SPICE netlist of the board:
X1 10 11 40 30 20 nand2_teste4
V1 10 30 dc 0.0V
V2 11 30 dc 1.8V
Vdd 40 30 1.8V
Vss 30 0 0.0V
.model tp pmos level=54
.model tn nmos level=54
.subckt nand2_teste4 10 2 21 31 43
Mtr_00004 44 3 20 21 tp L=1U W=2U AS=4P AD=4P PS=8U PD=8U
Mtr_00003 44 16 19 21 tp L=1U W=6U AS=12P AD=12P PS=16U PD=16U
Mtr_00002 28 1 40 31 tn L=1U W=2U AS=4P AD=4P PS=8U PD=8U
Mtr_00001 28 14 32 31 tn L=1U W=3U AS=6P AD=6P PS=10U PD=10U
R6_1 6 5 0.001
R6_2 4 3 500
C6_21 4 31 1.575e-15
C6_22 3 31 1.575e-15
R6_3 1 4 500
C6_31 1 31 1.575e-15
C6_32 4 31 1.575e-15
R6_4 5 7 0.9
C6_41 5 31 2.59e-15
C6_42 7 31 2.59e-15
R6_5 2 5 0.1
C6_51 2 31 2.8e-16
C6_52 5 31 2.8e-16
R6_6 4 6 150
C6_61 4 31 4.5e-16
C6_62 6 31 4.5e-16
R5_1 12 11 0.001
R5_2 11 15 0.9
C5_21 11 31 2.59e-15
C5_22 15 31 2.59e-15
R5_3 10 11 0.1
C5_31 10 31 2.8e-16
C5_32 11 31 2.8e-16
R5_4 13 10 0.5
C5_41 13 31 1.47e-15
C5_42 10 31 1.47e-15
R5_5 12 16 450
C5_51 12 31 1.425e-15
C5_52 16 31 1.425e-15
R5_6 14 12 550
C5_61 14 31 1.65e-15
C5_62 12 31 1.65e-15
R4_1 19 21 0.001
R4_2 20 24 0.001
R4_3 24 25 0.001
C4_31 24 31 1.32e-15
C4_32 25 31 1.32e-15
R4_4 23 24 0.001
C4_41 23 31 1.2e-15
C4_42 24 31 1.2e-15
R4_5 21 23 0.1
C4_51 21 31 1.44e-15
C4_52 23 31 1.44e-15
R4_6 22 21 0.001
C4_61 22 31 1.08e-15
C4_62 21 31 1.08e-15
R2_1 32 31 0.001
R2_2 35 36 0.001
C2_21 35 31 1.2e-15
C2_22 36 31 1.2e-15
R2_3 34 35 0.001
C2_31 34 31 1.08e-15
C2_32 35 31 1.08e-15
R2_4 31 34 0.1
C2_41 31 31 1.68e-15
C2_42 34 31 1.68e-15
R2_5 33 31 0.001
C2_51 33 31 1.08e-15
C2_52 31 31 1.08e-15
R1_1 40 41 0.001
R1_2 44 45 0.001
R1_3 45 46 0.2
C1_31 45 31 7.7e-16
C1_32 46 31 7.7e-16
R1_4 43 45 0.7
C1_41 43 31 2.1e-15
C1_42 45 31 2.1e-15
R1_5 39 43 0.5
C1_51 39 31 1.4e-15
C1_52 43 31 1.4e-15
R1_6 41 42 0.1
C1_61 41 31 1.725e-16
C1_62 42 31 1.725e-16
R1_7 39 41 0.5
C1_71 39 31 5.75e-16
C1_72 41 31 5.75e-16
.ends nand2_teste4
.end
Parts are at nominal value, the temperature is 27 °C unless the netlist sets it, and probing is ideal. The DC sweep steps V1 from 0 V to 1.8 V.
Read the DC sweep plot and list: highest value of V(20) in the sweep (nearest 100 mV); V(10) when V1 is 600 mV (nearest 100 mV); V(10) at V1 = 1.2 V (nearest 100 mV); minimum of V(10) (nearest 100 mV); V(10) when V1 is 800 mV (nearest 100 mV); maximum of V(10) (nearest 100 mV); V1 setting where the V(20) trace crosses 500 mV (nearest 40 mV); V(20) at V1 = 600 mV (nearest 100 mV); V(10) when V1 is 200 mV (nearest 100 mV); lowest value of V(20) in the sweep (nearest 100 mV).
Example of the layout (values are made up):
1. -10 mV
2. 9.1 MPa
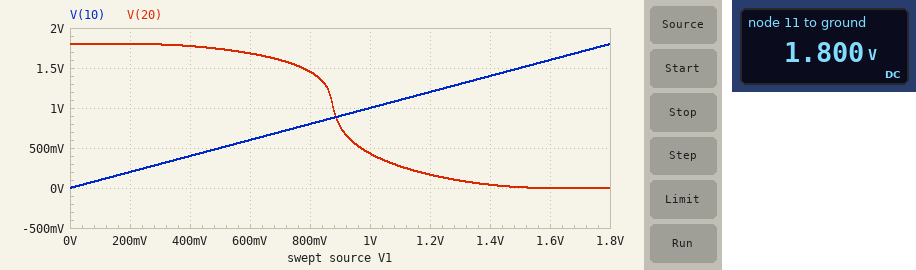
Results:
1. 1.8 V
2. 600 mV
3. 1.2 V
4. 0 V
5. 800 mV
6. 1.8 V
7. 960 mV
8. 1.7 V
9. 200 mV
10. 0 V
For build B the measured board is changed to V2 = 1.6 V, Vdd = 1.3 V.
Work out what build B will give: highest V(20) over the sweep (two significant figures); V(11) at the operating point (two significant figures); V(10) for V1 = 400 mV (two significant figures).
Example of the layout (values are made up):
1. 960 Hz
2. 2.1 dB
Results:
1. 1.3 V
2. 1.6 V
3. 400 mV
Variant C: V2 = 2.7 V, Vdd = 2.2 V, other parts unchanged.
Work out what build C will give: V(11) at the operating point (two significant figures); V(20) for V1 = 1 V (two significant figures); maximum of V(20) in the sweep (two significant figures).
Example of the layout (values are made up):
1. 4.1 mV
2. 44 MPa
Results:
1. 2.7 V
2. 1.7 V
3. 2.2 V
